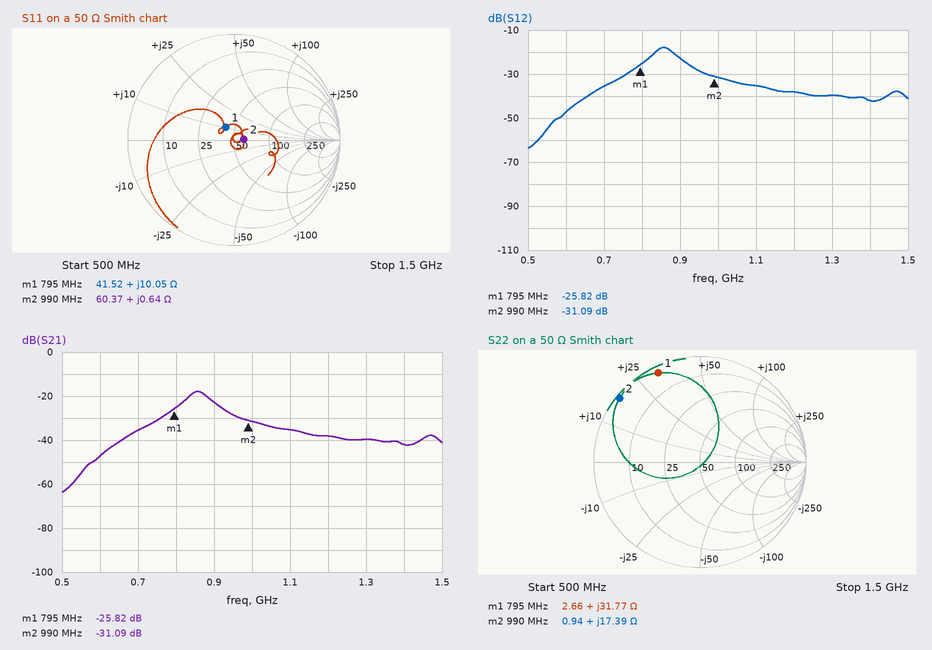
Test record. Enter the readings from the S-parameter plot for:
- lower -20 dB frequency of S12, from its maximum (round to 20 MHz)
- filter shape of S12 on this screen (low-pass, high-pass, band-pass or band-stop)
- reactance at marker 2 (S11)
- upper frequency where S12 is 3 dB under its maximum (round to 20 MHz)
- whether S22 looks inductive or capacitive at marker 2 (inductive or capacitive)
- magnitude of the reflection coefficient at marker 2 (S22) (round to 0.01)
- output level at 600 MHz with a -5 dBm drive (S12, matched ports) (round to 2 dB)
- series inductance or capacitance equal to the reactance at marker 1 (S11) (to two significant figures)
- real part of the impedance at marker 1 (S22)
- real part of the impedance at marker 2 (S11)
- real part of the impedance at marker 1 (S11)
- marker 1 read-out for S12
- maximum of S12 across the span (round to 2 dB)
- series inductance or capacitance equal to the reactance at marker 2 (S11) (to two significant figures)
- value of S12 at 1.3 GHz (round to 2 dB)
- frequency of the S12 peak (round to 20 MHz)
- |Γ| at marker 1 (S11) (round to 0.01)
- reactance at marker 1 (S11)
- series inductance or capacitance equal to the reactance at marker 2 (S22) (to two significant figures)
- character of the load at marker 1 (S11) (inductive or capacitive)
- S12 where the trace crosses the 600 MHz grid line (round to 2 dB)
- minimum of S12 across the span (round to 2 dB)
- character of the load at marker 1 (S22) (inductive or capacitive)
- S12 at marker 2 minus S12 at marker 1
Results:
680 MHz
band-pass
+0.64 Ω
880 MHz
inductive
0.97
-52 dBm
2.0 nH
2.66 Ω
60.37 Ω
41.52 Ω
-25.82 dB
-18 dB
100 pH
-40 dB
860 MHz
0.14
+10.05 Ω
2.8 nH
inductive
-48 dB
-64 dB
inductive
-5.27 dB
